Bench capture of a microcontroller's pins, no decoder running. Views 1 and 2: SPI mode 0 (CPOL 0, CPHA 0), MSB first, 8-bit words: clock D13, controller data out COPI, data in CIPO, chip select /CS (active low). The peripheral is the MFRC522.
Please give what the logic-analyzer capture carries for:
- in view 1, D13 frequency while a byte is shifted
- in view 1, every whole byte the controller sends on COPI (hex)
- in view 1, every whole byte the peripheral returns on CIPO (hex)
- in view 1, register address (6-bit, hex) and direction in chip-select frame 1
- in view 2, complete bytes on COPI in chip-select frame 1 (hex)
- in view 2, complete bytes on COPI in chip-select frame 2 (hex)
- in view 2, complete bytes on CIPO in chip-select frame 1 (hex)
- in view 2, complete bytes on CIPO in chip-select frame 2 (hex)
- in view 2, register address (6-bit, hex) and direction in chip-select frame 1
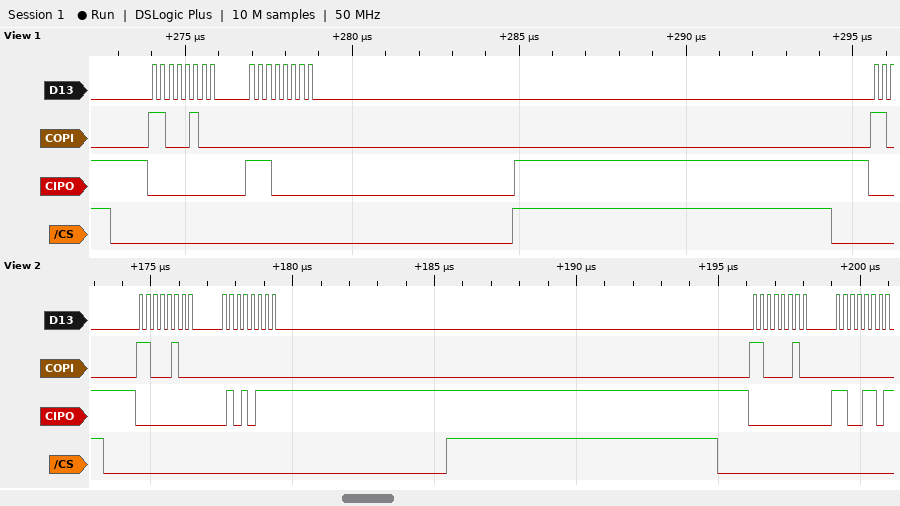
4 MHz
C4 00
00 E0
0x22 read
C4 00
C2 00
00 57
00 CD
0x22 read
